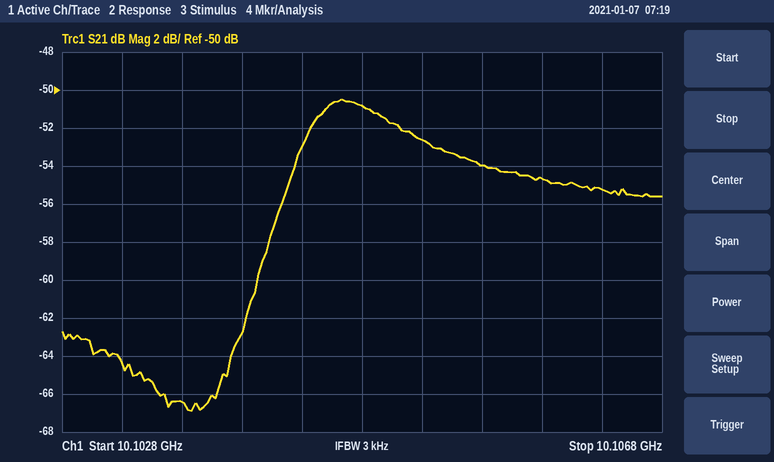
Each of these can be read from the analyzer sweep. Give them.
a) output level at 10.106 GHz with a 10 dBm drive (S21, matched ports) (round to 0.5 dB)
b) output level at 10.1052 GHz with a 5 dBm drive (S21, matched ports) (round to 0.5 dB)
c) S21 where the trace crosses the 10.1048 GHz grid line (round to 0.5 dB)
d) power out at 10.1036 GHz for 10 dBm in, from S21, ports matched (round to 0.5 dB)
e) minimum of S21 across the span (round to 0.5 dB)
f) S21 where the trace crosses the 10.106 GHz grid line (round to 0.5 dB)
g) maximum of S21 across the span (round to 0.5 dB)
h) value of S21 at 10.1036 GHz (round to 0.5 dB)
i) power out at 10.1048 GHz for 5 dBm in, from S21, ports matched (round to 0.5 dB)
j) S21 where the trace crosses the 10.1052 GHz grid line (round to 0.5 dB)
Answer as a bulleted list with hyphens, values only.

- -44.5 dBm
- -47.5 dBm
- -51.0 dB
- -56.5 dBm
- -67.0 dB
- -54.5 dB
- -50.5 dB
- -66.5 dB
- -46.0 dBm
- -52.5 dB
